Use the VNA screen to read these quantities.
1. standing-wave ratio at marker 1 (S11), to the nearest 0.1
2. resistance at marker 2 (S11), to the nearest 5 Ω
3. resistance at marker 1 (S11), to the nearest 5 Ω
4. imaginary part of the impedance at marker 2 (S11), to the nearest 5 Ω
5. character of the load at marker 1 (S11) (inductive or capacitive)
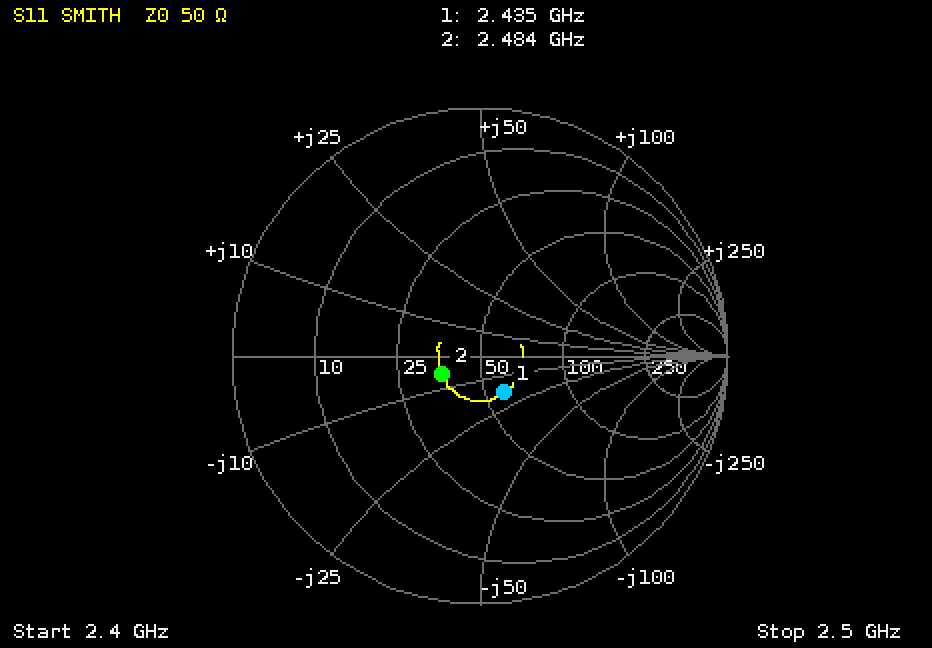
1.4
35 Ω
60 Ω
-5 Ω
capacitive
